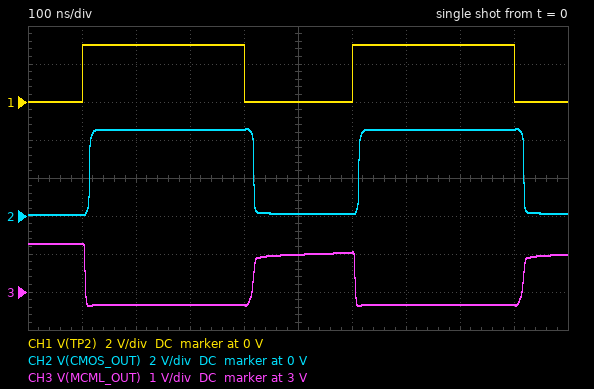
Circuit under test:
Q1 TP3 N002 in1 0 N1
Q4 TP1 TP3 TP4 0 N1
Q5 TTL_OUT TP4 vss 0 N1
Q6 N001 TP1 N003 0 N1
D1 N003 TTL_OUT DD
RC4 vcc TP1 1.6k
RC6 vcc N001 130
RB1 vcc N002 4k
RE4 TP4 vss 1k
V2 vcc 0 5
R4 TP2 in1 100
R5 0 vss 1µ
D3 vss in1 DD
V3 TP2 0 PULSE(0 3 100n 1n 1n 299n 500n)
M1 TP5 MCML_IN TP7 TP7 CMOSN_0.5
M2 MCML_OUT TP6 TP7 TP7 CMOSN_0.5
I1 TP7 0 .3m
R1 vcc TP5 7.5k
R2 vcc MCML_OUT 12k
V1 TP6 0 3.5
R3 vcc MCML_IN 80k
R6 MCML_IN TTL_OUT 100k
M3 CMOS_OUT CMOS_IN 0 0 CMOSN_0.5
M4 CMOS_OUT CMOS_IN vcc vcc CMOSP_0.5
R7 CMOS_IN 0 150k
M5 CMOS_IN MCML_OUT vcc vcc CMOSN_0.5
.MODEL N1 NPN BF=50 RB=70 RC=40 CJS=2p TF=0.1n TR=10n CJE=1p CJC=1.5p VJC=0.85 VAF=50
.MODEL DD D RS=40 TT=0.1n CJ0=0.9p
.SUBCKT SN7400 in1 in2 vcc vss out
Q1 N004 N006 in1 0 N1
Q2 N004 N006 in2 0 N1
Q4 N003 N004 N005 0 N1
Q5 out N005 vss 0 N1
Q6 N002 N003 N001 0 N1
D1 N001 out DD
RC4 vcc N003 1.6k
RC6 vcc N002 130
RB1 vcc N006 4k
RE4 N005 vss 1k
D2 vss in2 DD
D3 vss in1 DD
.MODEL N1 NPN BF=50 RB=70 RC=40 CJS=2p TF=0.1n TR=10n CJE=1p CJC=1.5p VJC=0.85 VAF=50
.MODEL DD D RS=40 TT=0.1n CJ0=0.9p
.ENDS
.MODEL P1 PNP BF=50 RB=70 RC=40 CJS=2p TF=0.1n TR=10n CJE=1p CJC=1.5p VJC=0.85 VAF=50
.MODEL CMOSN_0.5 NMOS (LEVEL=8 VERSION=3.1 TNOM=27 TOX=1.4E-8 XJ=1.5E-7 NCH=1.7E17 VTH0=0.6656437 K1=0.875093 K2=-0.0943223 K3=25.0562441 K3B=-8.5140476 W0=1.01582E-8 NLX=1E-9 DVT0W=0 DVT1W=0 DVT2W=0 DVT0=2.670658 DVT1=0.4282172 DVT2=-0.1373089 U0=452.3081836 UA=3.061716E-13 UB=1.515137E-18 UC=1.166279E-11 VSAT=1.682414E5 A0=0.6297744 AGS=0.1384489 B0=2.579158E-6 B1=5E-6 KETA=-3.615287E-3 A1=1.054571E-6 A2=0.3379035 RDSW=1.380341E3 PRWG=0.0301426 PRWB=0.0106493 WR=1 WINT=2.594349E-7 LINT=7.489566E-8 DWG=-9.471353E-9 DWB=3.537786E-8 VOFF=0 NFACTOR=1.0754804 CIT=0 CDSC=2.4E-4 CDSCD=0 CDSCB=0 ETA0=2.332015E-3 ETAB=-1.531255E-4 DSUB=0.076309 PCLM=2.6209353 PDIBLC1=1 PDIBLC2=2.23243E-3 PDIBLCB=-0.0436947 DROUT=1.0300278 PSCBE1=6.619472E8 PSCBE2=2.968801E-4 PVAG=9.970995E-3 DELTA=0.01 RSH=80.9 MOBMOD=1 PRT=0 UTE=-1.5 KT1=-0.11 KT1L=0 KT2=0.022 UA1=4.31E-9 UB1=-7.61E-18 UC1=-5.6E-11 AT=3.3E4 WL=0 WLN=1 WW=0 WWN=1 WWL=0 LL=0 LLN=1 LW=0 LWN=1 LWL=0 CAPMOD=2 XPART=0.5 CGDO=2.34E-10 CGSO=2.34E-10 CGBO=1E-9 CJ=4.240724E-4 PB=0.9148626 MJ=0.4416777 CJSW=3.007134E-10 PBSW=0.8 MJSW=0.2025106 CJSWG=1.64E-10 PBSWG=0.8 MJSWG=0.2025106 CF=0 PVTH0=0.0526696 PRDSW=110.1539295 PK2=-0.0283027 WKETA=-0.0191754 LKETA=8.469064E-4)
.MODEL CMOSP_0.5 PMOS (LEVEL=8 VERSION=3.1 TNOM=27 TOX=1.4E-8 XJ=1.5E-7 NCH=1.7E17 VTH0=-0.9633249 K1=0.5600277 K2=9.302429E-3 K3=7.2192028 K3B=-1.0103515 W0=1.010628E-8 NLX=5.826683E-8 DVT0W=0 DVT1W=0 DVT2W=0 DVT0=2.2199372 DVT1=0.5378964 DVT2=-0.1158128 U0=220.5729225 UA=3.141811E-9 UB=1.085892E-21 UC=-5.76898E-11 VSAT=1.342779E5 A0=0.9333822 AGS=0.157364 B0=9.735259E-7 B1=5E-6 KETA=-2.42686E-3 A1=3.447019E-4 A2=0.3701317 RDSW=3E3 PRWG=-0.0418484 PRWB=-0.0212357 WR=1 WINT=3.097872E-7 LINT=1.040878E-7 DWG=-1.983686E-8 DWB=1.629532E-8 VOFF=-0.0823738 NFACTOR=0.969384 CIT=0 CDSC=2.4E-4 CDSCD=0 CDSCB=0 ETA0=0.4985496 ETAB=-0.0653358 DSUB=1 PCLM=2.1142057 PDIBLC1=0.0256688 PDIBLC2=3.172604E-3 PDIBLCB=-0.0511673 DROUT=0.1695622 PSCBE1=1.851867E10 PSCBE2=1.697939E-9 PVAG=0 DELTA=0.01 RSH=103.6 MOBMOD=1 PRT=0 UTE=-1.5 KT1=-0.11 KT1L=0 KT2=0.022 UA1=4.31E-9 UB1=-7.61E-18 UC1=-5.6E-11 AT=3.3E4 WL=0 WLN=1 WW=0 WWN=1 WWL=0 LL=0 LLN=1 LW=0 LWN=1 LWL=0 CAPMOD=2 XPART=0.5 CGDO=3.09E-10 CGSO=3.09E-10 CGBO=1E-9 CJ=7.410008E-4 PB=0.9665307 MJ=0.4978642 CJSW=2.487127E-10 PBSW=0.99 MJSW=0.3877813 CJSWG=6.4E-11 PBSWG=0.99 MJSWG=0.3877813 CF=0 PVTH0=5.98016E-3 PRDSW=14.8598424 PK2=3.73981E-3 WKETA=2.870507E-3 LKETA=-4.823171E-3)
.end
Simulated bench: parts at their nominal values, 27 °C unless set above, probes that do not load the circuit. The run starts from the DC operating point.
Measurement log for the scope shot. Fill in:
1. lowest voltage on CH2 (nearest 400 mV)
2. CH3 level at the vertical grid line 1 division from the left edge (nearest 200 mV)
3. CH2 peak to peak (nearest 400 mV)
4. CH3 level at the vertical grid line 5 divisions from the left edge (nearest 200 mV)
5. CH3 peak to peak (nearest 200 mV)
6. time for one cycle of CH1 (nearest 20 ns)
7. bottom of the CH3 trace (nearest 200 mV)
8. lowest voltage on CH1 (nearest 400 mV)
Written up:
0 V
4.2 V
4.4 V
4.0 V
1.6 V
500 ns
2.6 V
0 V
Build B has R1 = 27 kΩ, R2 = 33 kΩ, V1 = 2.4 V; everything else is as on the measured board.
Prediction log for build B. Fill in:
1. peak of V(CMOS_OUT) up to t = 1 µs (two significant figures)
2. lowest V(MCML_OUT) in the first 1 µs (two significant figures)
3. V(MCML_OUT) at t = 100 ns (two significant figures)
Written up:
5.0 V
470 mV
870 mV
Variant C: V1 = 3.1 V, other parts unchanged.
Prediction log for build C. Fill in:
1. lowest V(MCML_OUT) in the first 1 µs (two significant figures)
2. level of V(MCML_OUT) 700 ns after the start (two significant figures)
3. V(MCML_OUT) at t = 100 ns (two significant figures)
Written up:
2.9 V
3.0 V
4.5 V
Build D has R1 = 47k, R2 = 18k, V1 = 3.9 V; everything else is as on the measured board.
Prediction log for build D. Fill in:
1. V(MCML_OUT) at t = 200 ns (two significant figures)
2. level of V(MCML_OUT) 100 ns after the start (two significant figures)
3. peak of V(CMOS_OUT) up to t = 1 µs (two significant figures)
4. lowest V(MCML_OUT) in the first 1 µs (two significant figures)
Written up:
1.2 V
1.3 V
5.0 V
1.0 V
